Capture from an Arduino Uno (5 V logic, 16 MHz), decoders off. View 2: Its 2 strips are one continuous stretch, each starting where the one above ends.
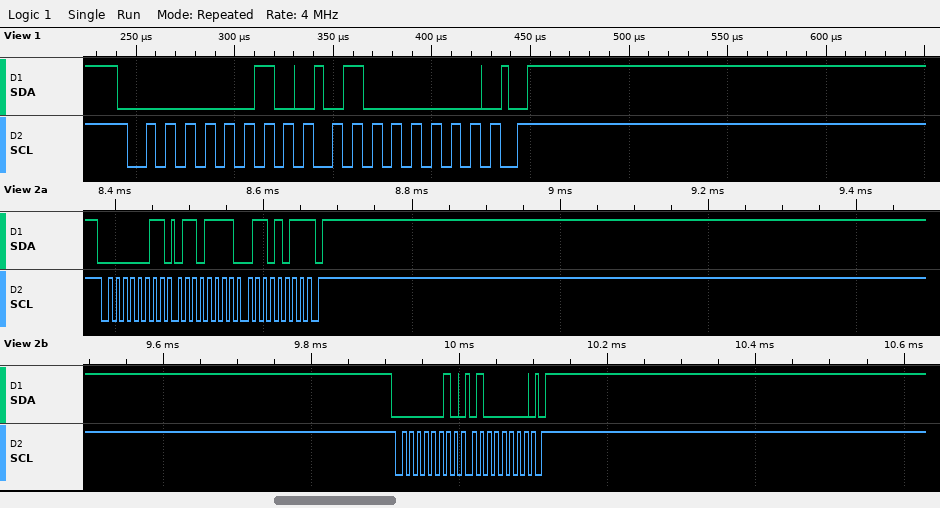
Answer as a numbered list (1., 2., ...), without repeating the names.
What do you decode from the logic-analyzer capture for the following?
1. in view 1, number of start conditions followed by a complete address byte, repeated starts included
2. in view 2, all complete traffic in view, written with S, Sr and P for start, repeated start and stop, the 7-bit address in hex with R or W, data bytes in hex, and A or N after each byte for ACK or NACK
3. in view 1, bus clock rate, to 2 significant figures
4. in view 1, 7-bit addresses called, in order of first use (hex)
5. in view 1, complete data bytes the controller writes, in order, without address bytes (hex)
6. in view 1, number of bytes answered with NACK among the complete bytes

1. 1
2. S 01R A 6F A 6B N P S 01W A 40 A P
3. 100 kHz
4. 0x01
5. 40
6. 0
